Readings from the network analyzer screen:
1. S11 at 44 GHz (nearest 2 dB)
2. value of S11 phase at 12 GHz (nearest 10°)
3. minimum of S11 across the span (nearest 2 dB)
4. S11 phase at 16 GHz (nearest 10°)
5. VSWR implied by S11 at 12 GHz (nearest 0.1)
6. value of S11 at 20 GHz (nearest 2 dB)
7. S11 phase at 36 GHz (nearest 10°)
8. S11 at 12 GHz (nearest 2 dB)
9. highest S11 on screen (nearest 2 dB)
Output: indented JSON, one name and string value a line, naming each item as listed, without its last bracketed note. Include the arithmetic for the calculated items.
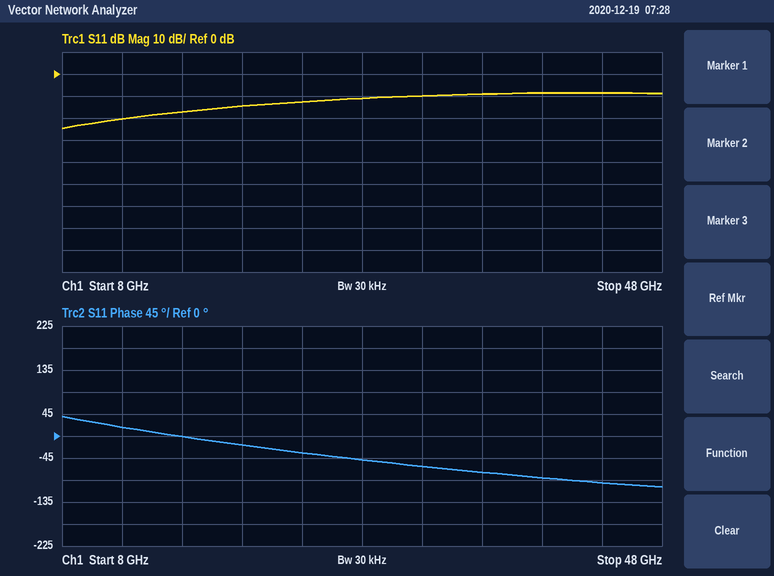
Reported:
{
  "S11 at 44 GHz": "-8 dB",
  "value of S11 phase at 12 GHz": "20°",
  "minimum of S11 across the span": "-24 dB",
  "S11 phase at 16 GHz": "0°",
  "VSWR implied by S11 at 12 GHz": "|Γ| = 10^(-20/20) = 0.1000; VSWR = (1 + 0.1000)/(1 − 0.1000) ≈ 1.2",
  "value of S11 at 20 GHz": "-14 dB",
  "S11 phase at 36 GHz": "-70°",
  "S11 at 12 GHz": "-20 dB",
  "highest S11 on screen": "-8 dB"
}
